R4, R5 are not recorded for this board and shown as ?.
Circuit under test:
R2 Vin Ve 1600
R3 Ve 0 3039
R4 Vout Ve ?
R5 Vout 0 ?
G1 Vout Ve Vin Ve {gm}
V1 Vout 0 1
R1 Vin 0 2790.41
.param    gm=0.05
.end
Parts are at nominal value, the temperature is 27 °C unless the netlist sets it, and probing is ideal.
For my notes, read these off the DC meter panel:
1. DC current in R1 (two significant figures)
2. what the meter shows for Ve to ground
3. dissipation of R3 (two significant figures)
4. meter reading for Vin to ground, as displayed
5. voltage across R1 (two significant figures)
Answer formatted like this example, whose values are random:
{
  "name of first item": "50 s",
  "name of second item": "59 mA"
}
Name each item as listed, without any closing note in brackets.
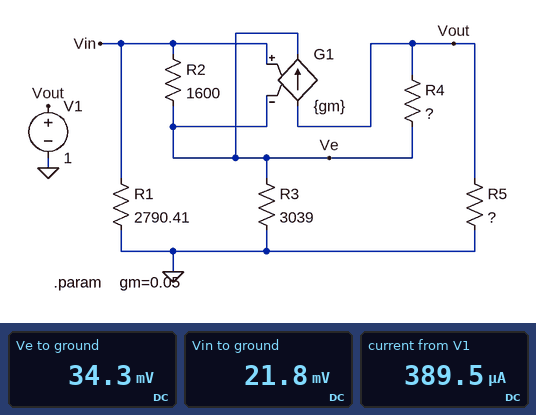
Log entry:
{
  "DC current in R1": "7.8 µA",
  "what the meter shows for Ve to ground": "34.3 mV",
  "dissipation of R3": "390 nW",
  "meter reading for Vin to ground, as displayed": "21.8 mV",
  "voltage across R1": "22 mV"
}
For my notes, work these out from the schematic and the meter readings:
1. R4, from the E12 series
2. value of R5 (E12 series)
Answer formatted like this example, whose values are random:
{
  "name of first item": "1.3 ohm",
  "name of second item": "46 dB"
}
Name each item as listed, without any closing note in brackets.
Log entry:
{
  "R4, from the E12 series": "1.5 kΩ",
  "value of R5": "2.7 kΩ"
}
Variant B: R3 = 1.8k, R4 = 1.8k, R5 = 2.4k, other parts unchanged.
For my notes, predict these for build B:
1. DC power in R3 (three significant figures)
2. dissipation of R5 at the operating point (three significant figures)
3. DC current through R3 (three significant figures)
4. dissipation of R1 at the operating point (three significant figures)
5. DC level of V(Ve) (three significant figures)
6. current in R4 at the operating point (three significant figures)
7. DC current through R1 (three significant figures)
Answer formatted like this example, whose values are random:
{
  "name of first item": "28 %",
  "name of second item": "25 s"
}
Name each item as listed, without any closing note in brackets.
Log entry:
{
  "DC power in R3": "448 nW",
  "dissipation of R5 at the operating point": "417 µW",
  "DC current through R3": "15.8 µA",
  "dissipation of R1 at the operating point": "117 nW",
  "DC level of V(Ve)": "28.4 mV",
  "current in R4 at the operating point": "540 µA",
  "DC current through R1": "6.47 µA"
}
